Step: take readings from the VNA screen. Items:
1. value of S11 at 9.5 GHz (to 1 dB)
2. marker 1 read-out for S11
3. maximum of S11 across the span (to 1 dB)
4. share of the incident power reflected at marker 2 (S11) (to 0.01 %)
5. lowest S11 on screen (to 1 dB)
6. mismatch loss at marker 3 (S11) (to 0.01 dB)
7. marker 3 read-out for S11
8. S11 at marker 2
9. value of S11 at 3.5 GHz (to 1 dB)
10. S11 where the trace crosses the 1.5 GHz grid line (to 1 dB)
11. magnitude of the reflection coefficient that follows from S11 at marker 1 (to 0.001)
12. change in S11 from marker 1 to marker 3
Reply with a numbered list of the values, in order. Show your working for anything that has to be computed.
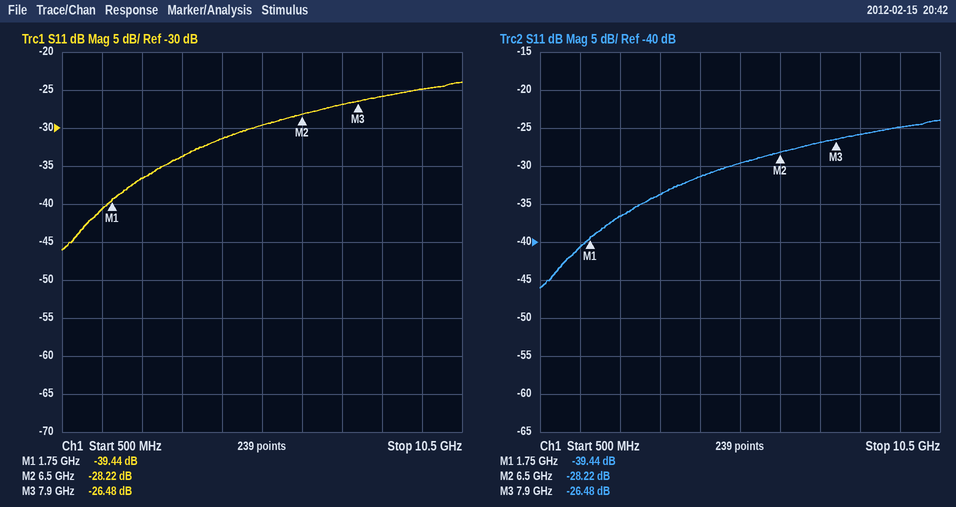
1. -25 dB
2. -39.44 dB
3. -24 dB
4. 10^(-28.22/10) ≈ 0.15 %
5. -46 dB
6. −10 log10(1 − 10^(-26.48/10)) ≈ 0.01 dB
7. -26.48 dB
8. -28.22 dB
9. -34 dB
10. -41 dB
11. 10^(-39.44/20) ≈ 0.011
12. -26.48 − (-39.44) = 12.96 dB
